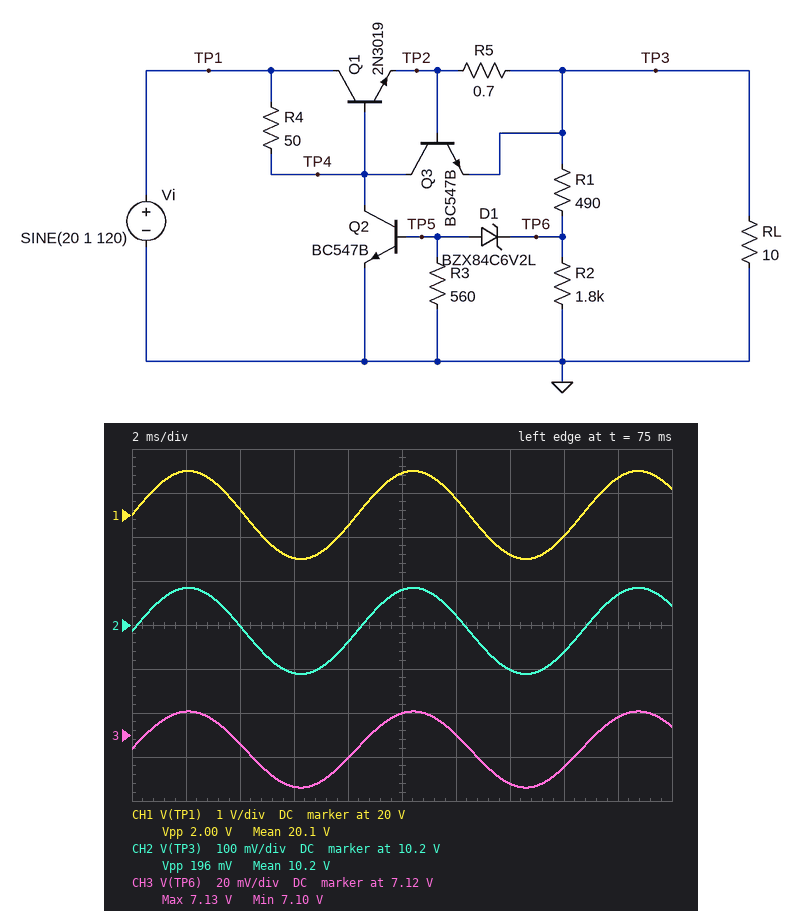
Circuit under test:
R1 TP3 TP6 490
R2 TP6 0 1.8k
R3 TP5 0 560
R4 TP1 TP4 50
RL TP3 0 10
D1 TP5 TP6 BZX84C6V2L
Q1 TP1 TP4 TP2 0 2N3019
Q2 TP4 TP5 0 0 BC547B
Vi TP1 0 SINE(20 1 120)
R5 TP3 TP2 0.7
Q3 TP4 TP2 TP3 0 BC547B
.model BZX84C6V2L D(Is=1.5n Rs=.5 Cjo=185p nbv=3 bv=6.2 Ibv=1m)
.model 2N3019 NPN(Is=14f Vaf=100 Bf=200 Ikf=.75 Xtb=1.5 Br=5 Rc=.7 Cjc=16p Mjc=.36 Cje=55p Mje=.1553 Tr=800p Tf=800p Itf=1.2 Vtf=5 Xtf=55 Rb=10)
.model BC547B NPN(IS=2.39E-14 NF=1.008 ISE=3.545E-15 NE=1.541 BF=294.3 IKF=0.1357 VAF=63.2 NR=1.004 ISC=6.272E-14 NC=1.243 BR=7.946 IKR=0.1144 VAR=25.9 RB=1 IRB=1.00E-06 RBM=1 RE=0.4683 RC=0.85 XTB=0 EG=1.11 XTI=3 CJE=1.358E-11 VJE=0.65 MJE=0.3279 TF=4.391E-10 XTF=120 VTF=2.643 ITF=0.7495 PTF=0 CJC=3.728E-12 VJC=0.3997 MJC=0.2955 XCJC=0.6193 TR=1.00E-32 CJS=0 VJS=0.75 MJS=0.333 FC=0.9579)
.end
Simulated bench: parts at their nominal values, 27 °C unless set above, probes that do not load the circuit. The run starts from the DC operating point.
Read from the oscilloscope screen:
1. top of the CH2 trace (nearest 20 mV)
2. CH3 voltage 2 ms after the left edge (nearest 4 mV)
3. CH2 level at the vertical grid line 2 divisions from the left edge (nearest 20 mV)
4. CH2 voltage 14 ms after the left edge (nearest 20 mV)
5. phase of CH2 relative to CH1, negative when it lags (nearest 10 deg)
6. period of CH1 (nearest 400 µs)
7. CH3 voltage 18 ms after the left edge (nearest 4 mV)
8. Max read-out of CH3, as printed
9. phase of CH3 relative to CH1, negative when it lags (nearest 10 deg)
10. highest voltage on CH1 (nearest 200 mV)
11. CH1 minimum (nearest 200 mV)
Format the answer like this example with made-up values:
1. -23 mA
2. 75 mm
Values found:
1. 10.28 V
2. 7.132 V
3. 10.20 V
4. 10.10 V
5. 0 deg
6. 8.4 ms
7. 7.128 V
8. 7.13 V
9. 0 deg
10. 21.0 V
11. 19.0 V
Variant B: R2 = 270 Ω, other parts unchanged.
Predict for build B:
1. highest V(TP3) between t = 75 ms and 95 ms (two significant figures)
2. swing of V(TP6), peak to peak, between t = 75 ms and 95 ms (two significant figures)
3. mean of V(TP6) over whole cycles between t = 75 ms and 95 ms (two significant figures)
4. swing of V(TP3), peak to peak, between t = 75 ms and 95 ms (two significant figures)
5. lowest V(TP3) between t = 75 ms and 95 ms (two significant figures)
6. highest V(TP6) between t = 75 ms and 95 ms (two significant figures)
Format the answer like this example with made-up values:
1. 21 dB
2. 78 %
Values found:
1. 13 V
2. 210 mV
3. 4.5 V
4. 600 mV
5. 12 V
6. 4.6 V
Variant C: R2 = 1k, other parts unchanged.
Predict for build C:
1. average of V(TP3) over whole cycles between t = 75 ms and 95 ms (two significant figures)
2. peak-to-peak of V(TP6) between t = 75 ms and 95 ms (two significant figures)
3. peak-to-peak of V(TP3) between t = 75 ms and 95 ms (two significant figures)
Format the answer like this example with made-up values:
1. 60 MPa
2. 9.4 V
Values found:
1. 11 V
2. 38 mV
3. 170 mV
